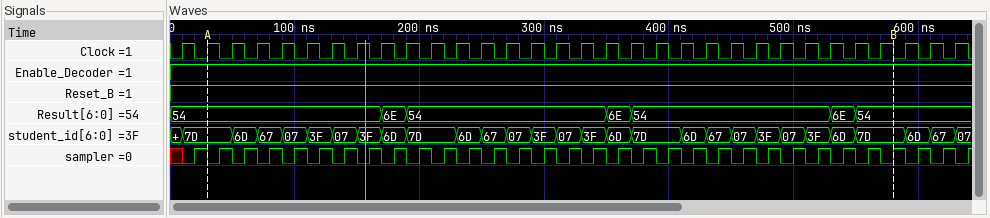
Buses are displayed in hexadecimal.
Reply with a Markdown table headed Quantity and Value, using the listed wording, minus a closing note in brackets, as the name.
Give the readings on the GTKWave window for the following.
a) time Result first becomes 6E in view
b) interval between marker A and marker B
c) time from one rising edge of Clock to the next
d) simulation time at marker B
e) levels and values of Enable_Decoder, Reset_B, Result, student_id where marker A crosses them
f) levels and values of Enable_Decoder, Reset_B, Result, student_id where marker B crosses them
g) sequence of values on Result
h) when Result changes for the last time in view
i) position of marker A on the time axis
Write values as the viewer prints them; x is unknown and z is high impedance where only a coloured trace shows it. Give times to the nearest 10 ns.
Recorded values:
| Quantity | Value |
|---|---|
| time Result first becomes 6E in view | 170 ns |
| interval between marker A and marker B | 550 ns |
| time from one rising edge of Clock to the next | 20 ns |
| simulation time at marker B | 580 ns |
| levels and values of Enable_Decoder, Reset_B, Result, student_id where marker A crosses them | Enable_Decoder=1, Reset_B=1, Result=54, student_id=7D |
| levels and values of Enable_Decoder, Reset_B, Result, student_id where marker B crosses them | Enable_Decoder=1, Reset_B=1, Result=54, student_id=7D |
| sequence of values on Result | 54, 6E, 54, 6E, 54, 6E, 54 |
| when Result changes for the last time in view | 550 ns |
| position of marker A on the time axis | 30 ns |
